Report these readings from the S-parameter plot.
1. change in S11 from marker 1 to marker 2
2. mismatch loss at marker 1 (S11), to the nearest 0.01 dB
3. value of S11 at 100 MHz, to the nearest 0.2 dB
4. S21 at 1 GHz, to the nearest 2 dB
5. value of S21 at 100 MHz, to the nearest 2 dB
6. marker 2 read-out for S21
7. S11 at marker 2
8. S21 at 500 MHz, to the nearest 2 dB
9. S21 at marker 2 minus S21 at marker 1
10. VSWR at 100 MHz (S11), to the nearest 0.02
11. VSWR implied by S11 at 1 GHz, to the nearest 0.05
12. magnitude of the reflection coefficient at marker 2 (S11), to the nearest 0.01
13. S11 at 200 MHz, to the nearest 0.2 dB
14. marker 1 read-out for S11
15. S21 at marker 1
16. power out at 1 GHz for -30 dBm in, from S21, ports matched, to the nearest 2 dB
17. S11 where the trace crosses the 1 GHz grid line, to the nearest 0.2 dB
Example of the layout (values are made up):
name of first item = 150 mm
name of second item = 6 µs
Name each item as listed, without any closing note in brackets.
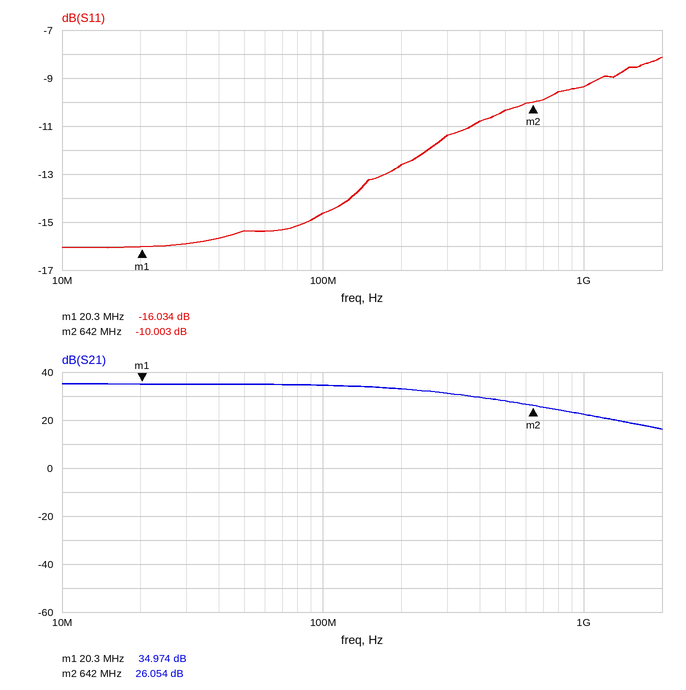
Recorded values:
change in S11 from marker 1 to marker 2 = 6.031 dB
mismatch loss at marker 1 (S11), to the nearest 0.01 dB = 0.11 dB
value of S11 at 100 MHz, to the nearest 0.2 dB = -14.6 dB
S21 at 1 GHz, to the nearest 2 dB = 22 dB
value of S21 at 100 MHz, to the nearest 2 dB = 34 dB
marker 2 read-out for S21 = 26.054 dB
S11 at marker 2 = -10.003 dB
S21 at 500 MHz, to the nearest 2 dB = 28 dB
S21 at marker 2 minus S21 at marker 1 = -8.920 dB
VSWR at 100 MHz (S11), to the nearest 0.02 = 1.46
VSWR implied by S11 at 1 GHz, to the nearest 0.05 = 2.05
magnitude of the reflection coefficient at marker 2 (S11), to the nearest 0.01 = 0.32
S11 at 200 MHz, to the nearest 0.2 dB = -12.6 dB
marker 1 read-out for S11 = -16.034 dB
S21 at marker 1 = 34.974 dB
power out at 1 GHz for -30 dBm in, from S21, ports matched, to the nearest 2 dB = -8 dBm
S11 where the trace crosses the 1 GHz grid line, to the nearest 0.2 dB = -9.4 dB
